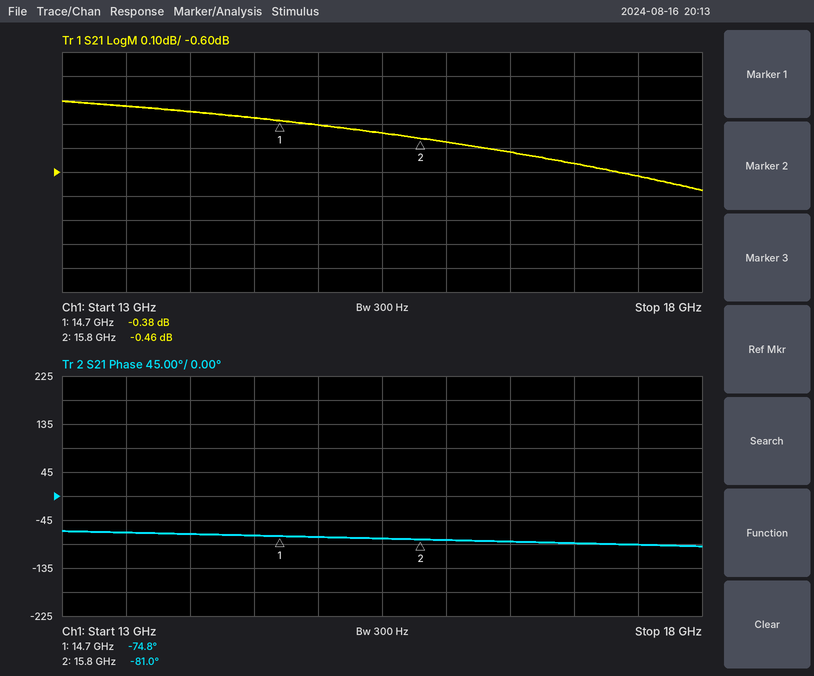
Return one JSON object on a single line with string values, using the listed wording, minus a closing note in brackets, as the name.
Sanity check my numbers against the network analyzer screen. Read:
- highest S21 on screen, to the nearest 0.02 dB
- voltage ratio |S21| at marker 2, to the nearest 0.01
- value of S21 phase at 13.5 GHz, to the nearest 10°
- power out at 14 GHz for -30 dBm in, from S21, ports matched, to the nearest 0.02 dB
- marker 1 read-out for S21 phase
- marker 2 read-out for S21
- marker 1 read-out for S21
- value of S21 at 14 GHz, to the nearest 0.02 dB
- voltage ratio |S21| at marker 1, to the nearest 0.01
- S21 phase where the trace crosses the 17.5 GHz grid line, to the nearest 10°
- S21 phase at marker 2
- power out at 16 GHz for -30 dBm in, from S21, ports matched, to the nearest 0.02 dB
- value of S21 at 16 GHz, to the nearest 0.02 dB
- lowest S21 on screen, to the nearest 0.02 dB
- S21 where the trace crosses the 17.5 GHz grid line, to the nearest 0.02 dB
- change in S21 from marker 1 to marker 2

{"highest S21 on screen, to the nearest 0.02 dB": "-0.30 dB", "voltage ratio |S21| at marker 2, to the nearest 0.01": "0.95", "value of S21 phase at 13.5 GHz, to the nearest 10°": "-70°", "power out at 14 GHz for -30 dBm in, from S21, ports matched, to the nearest 0.02 dB": "-30.34 dBm", "marker 1 read-out for S21 phase": "-74.8°", "marker 2 read-out for S21": "-0.46 dB", "marker 1 read-out for S21": "-0.38 dB", "value of S21 at 14 GHz, to the nearest 0.02 dB": "-0.34 dB", "voltage ratio |S21| at marker 1, to the nearest 0.01": "0.96", "S21 phase where the trace crosses the 17.5 GHz grid line, to the nearest 10°": "-90°", "S21 phase at marker 2": "-81.0°", "power out at 16 GHz for -30 dBm in, from S21, ports matched, to the nearest 0.02 dB": "-30.48 dBm", "value of S21 at 16 GHz, to the nearest 0.02 dB": "-0.48 dB", "lowest S21 on screen, to the nearest 0.02 dB": "-0.68 dB", "S21 where the trace crosses the 17.5 GHz grid line, to the nearest 0.02 dB": "-0.62 dB", "change in S21 from marker 1 to marker 2": "-0.08 dB"}
